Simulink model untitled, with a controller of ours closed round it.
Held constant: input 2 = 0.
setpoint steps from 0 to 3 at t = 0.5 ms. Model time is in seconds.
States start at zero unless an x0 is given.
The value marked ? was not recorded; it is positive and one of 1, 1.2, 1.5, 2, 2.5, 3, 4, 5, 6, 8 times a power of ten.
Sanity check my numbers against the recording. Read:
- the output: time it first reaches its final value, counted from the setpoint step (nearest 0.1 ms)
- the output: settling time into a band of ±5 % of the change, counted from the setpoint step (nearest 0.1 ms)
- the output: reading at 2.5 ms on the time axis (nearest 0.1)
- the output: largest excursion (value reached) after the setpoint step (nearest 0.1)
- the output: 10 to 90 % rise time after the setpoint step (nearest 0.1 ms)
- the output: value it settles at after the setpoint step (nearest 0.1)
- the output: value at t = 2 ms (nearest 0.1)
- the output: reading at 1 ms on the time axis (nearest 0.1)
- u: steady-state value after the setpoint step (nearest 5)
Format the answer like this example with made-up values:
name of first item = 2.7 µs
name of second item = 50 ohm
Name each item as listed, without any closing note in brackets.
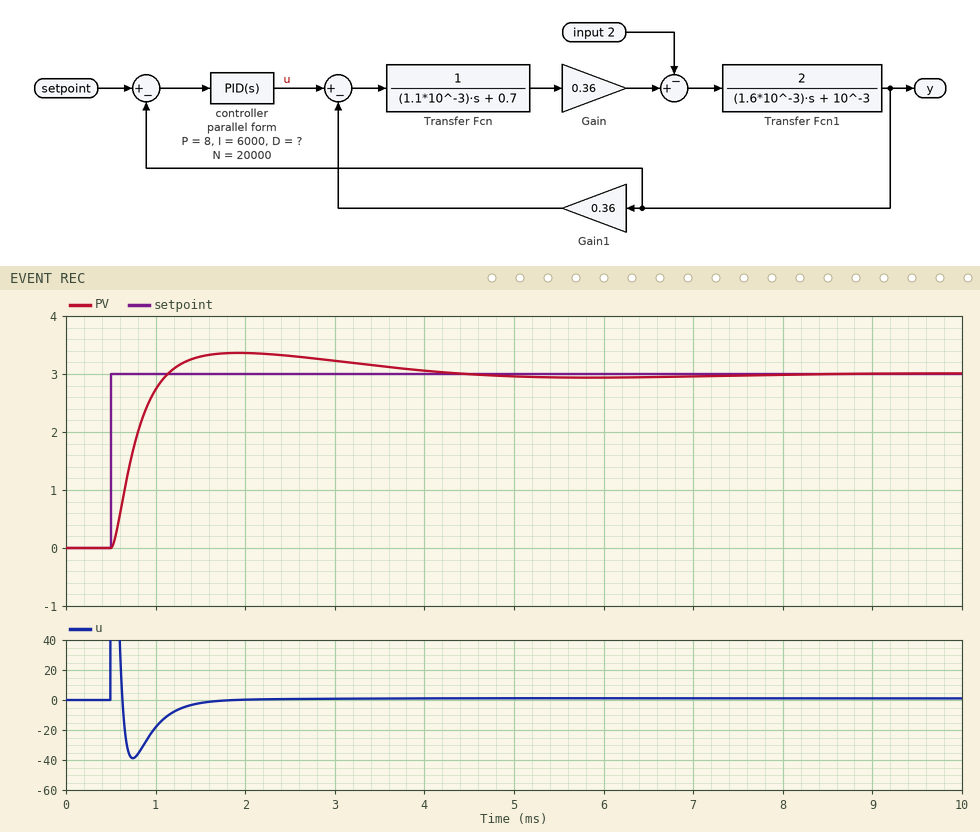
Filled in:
the output: time it first reaches its final value, counted from the setpoint step = 0.6 ms
the output: settling time into a band of ±5 % of the change, counted from the setpoint step = 2.9 ms
the output: reading at 2.5 ms on the time axis = 3.3
the output: largest excursion (value reached) after the setpoint step = 3.4
the output: 10 to 90 % rise time after the setpoint step = 0.4 ms
the output: value it settles at after the setpoint step = 3.0
the output: value at t = 2 ms = 3.4
the output: reading at 1 ms on the time axis = 2.7
u: steady-state value after the setpoint step = 0
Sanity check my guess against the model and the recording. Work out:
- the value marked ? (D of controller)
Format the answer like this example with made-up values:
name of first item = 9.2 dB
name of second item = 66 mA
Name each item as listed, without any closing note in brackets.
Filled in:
the value marked ? = 0.008
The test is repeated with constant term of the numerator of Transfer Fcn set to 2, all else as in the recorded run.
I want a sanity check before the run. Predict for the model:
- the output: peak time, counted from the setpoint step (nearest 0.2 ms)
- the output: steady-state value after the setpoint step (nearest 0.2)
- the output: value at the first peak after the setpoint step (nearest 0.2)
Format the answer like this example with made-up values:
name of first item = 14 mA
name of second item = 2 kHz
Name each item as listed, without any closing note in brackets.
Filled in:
the output: peak time, counted from the setpoint step = 0.6 ms
the output: steady-state value after the setpoint step = 3.0
the output: value at the first peak after the setpoint step = 3.2
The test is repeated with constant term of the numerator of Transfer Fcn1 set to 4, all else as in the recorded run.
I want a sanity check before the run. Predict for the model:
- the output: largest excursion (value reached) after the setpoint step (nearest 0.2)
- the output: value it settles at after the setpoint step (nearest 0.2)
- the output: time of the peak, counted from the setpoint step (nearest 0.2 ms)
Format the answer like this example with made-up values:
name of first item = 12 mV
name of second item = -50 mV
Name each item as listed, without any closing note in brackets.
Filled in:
the output: largest excursion (value reached) after the setpoint step = 3.2
the output: value it settles at after the setpoint step = 3.0
the output: time of the peak, counted from the setpoint step = 0.6 ms
